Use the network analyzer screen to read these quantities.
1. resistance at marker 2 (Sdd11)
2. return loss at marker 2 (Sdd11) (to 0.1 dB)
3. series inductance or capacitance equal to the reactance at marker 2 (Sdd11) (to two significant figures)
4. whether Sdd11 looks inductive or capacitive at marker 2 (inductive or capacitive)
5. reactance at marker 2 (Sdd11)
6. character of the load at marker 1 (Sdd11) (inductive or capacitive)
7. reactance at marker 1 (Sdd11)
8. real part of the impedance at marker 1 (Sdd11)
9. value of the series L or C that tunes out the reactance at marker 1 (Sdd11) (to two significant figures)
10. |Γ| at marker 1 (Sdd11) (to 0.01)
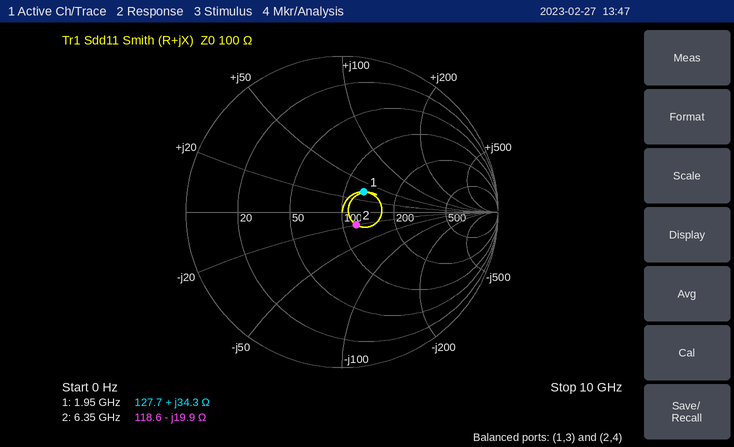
118.6 Ω
18.1 dB
1.3 pF
capacitive
-19.9 Ω
inductive
+34.3 Ω
127.7 Ω
2.4 pF
0.19
